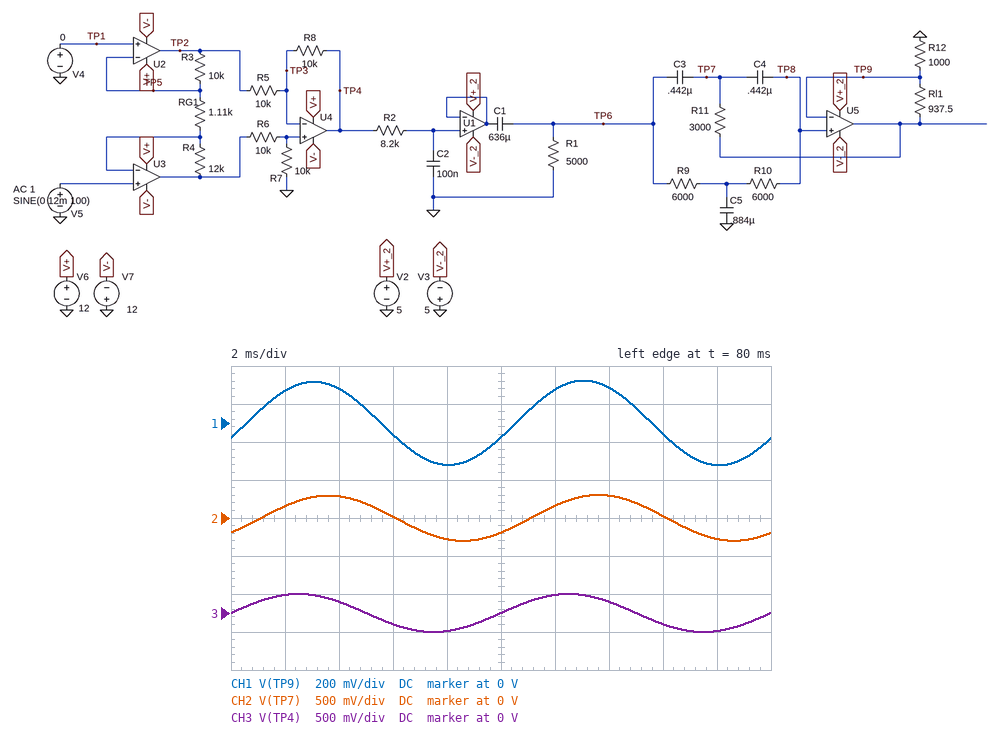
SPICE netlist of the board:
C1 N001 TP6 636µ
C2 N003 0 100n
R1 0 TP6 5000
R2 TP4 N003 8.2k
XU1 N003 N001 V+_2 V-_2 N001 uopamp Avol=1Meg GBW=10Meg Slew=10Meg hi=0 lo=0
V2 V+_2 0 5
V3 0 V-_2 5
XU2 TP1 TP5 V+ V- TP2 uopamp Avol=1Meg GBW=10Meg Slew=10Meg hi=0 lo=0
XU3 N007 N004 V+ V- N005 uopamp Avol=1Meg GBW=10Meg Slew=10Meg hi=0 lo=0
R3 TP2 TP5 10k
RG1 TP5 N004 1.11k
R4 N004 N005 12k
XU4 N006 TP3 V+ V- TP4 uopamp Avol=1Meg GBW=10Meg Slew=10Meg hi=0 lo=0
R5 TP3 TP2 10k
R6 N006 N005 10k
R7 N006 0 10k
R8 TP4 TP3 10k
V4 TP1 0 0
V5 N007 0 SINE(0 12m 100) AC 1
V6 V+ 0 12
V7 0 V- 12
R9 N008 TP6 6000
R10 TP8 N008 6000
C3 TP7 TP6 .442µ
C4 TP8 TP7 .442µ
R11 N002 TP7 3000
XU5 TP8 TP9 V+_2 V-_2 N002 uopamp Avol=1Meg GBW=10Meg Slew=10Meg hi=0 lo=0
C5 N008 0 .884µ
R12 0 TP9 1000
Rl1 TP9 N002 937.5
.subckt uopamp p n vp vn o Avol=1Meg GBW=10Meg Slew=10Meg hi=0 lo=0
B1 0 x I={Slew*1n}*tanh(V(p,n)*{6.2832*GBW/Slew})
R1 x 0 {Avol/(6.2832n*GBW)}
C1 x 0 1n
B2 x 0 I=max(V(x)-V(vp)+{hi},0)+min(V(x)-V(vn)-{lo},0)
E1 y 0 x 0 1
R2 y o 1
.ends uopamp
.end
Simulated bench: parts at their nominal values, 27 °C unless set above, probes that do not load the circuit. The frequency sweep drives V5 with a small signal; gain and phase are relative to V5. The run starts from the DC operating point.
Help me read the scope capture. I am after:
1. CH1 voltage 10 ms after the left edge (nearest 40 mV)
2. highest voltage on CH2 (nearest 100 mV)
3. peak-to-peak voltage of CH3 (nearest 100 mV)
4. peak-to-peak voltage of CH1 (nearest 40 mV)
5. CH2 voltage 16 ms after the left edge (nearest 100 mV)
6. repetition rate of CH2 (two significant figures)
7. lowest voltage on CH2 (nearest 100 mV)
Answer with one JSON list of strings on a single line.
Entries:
["-80 mV", "300 mV", "500 mV", "440 mV", "0 V", "100 Hz", "-300 mV"]
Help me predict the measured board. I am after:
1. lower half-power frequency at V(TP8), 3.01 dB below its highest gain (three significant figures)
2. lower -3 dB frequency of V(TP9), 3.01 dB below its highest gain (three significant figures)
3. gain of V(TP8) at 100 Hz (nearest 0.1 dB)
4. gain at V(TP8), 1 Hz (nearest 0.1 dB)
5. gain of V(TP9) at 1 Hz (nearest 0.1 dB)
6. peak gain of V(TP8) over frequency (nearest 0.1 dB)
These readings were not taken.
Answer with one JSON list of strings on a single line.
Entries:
["50.0 mHz", "50.0 mHz", "25.3 dB", "26.4 dB", "26.4 dB", "26.4 dB"]
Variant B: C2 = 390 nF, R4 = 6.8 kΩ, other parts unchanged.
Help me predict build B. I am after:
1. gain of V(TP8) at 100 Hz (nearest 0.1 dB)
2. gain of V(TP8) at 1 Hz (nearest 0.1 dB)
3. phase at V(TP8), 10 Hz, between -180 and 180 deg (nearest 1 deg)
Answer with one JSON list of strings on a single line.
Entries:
["17.1 dB", "24.1 dB", "-12 deg"]
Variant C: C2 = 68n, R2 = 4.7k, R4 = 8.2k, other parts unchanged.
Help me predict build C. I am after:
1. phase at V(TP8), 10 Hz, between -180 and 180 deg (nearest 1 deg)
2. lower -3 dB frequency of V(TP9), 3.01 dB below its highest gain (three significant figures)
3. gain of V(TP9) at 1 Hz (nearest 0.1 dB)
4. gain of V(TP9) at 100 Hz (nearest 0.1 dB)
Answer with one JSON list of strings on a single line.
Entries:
["-2 deg", "50.0 mHz", "24.8 dB", "24.6 dB"]
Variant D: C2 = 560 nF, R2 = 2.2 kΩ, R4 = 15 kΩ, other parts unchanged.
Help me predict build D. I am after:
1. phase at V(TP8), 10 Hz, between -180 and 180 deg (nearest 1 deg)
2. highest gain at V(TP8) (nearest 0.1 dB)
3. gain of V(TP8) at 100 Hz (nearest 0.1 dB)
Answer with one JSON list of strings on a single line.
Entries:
["-5 deg", "27.4 dB", "25.3 dB"]
